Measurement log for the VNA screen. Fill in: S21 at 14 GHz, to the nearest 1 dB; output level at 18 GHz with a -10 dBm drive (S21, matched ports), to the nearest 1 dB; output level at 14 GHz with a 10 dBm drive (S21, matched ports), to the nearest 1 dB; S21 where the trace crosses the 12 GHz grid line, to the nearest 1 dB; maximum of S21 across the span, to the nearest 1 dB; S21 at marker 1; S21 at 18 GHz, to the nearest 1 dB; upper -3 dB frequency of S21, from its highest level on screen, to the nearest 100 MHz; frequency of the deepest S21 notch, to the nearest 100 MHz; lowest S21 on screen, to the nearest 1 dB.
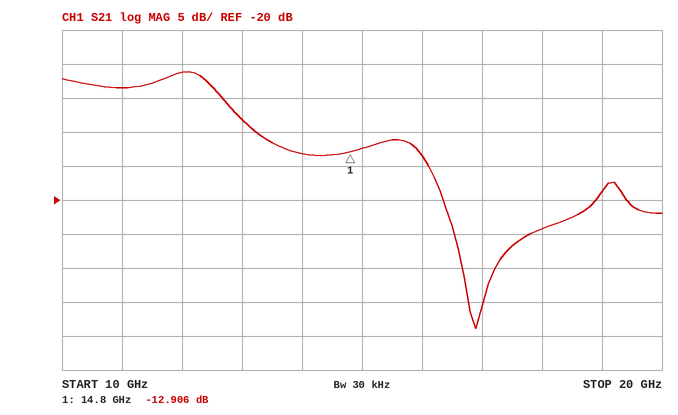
-13 dB
-34 dBm
-3 dBm
-1 dB
-1 dB
-12.906 dB
-24 dB
12.6 GHz
16.9 GHz
-39 dB
